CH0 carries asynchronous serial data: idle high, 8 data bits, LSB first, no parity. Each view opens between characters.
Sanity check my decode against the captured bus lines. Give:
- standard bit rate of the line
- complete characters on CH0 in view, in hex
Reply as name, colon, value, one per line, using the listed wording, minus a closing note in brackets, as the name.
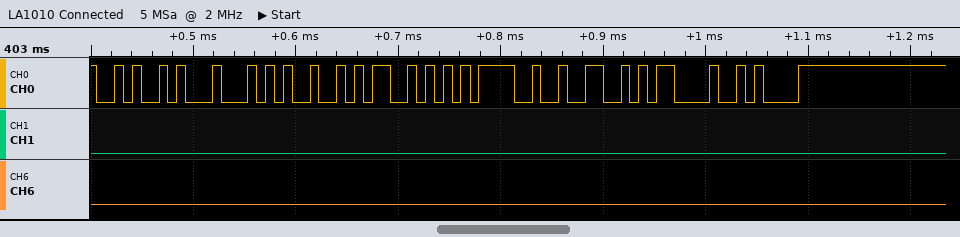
standard bit rate of the line: 115200 baud
complete characters on CH0 in view, in hex: 4A, 44, 49, 53, 3D, 32, 0D, 0A
